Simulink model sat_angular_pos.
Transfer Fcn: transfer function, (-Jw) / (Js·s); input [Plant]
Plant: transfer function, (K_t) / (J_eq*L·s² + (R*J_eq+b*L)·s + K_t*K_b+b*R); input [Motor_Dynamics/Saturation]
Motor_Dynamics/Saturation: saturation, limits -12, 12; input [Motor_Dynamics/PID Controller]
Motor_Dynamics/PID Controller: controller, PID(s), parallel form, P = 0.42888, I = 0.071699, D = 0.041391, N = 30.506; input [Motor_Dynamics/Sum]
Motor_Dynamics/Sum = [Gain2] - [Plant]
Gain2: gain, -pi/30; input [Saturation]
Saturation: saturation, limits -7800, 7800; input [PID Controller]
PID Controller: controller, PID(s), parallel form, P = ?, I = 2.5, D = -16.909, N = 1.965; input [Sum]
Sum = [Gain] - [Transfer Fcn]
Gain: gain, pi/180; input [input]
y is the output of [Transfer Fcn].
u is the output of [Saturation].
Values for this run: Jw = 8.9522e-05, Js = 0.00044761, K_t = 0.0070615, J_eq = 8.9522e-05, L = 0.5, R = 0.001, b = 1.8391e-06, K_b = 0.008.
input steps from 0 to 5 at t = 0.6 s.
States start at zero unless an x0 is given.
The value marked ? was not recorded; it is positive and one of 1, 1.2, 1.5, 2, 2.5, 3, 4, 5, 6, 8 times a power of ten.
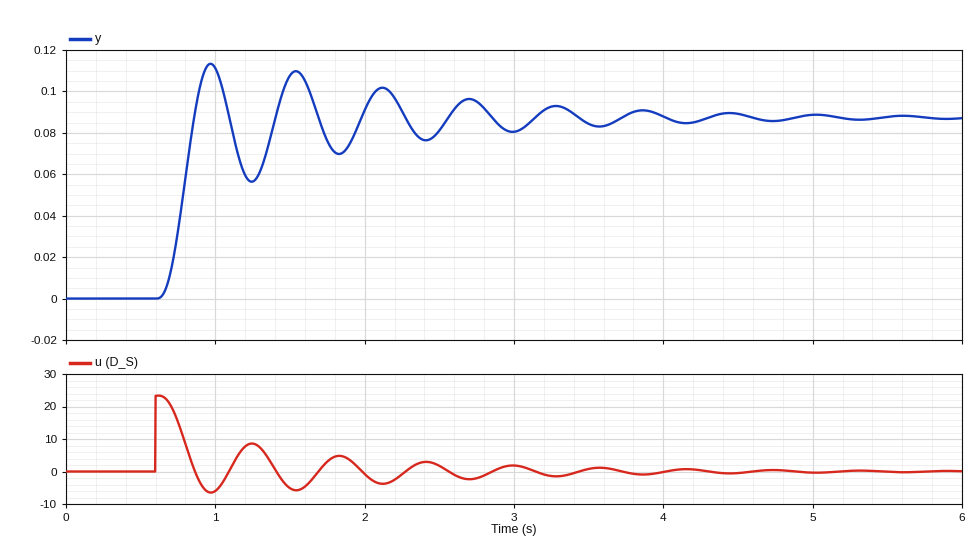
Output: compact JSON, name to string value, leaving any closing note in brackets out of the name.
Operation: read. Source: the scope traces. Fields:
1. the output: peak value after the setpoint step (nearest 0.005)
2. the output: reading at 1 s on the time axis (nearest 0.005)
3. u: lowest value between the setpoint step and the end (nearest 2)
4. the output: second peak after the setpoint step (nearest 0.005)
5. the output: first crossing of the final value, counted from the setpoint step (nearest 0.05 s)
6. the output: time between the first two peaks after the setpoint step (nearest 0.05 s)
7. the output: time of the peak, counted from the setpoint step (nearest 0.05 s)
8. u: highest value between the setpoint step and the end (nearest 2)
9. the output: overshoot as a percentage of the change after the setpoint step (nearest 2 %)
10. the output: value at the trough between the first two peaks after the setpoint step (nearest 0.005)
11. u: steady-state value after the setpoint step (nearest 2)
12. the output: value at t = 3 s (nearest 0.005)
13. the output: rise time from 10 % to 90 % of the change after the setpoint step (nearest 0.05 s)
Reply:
{"the output: peak value after the setpoint step": "0.115", "the output: reading at 1 s on the time axis": "0.110", "u: lowest value between the setpoint step and the end": "-6", "the output: second peak after the setpoint step": "0.110", "the output: first crossing of the final value, counted from the setpoint step": "0.25 s", "the output: time between the first two peaks after the setpoint step": "0.55 s", "the output: time of the peak, counted from the setpoint step": "0.35 s", "u: highest value between the setpoint step and the end": "24", "the output: overshoot as a percentage of the change after the setpoint step": "30 %", "the output: value at the trough between the first two peaks after the setpoint step": "0.055", "u: steady-state value after the setpoint step": "0", "the output: value at t = 3 s": "0.080", "the output: rise time from 10 % to 90 % of the change after the setpoint step": "0.15 s"}
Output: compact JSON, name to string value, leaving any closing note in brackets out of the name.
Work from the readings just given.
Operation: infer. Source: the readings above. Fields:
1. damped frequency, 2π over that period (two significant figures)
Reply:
{"damped frequency, 2π over that period": "11 rad/s"}
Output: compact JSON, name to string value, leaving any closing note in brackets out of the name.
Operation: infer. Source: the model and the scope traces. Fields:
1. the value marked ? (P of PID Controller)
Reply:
{"the value marked ?": "300"}
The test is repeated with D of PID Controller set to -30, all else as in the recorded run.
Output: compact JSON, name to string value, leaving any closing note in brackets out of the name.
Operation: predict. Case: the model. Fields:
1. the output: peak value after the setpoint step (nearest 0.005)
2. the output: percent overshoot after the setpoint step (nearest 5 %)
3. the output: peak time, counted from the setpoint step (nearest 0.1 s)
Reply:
{"the output: peak value after the setpoint step": "0.110", "the output: percent overshoot after the setpoint step": "25 %", "the output: peak time, counted from the setpoint step": "0.4 s"}
